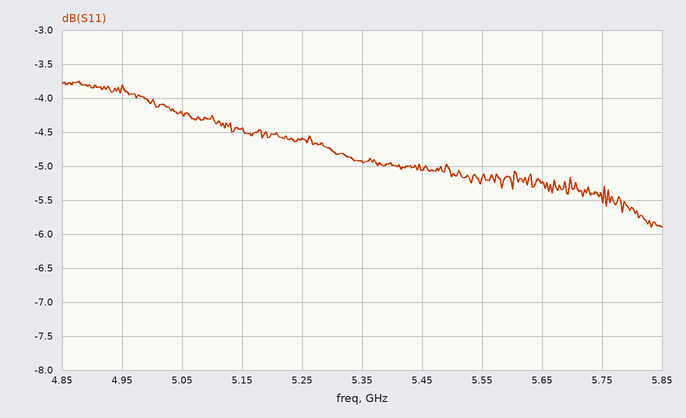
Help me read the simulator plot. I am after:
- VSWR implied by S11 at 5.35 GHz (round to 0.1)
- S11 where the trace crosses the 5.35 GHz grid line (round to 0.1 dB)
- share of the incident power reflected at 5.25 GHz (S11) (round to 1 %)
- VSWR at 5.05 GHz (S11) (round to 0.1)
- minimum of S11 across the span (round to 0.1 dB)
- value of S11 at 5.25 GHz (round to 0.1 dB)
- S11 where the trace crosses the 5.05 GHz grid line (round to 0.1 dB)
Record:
3.6
-4.9 dB
35 %
4.2
-5.9 dB
-4.6 dB
-4.2 dB
